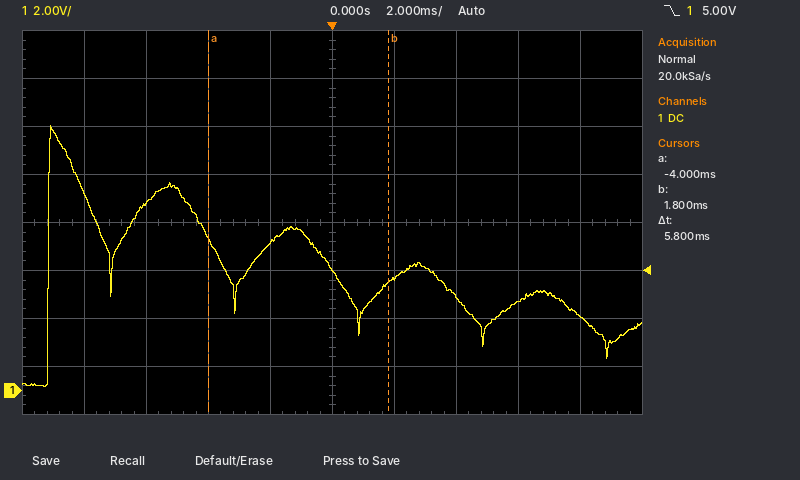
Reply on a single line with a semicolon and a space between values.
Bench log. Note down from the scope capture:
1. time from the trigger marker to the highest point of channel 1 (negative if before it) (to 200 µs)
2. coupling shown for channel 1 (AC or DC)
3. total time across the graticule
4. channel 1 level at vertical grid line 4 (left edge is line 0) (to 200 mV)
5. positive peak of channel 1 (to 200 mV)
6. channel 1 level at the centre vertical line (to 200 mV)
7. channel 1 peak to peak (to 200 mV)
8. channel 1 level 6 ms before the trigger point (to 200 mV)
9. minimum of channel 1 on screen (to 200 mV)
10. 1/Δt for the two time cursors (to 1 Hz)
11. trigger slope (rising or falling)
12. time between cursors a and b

-9.0 ms; DC; 20 ms; 6.2 V; 11.0 V; 5.0 V; 10.8 V; 7.8 V; 200 mV; 172 Hz; falling; 5.8 ms
